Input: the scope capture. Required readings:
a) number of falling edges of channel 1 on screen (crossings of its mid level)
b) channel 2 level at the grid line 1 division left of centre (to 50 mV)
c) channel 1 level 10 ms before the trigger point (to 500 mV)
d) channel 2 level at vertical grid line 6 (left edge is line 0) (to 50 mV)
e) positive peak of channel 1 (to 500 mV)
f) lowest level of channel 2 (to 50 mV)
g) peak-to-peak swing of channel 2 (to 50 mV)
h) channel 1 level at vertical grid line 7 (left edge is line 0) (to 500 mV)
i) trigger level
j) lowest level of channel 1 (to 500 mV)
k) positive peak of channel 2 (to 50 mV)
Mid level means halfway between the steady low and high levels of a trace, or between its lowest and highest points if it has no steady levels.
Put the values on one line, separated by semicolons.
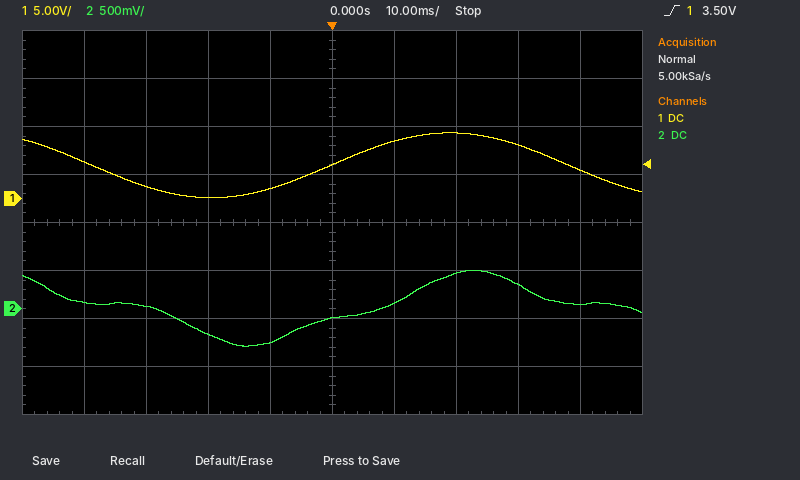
2; -350 mV; 1.0 V; 50 mV; 7.0 V; -400 mV; 800 mV; 7.0 V; 3.50 V; 0.0 V; 400 mV
